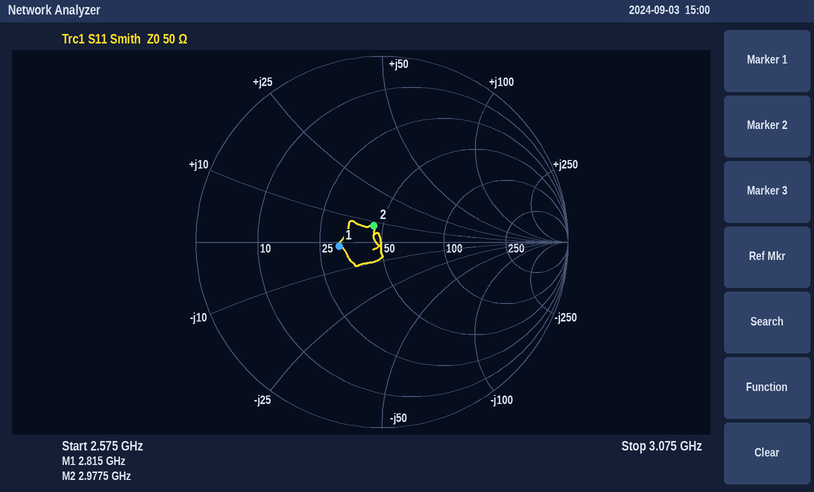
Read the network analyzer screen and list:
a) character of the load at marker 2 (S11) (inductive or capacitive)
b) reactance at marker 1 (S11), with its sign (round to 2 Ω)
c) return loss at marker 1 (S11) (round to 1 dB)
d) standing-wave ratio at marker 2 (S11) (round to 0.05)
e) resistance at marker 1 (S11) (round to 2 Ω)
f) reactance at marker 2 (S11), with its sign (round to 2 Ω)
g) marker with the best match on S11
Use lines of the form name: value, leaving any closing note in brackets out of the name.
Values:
character of the load at marker 2 (S11): inductive
reactance at marker 1 (S11), with its sign: -2 Ω
return loss at marker 1 (S11): 13 dB
standing-wave ratio at marker 2 (S11): 1.20
resistance at marker 1 (S11): 32 Ω
reactance at marker 2 (S11), with its sign: +8 Ω
marker with the best match on S11: marker 2
